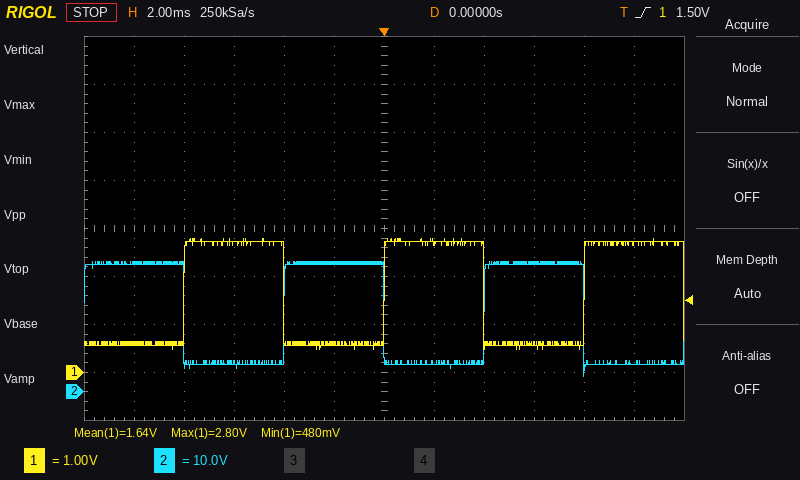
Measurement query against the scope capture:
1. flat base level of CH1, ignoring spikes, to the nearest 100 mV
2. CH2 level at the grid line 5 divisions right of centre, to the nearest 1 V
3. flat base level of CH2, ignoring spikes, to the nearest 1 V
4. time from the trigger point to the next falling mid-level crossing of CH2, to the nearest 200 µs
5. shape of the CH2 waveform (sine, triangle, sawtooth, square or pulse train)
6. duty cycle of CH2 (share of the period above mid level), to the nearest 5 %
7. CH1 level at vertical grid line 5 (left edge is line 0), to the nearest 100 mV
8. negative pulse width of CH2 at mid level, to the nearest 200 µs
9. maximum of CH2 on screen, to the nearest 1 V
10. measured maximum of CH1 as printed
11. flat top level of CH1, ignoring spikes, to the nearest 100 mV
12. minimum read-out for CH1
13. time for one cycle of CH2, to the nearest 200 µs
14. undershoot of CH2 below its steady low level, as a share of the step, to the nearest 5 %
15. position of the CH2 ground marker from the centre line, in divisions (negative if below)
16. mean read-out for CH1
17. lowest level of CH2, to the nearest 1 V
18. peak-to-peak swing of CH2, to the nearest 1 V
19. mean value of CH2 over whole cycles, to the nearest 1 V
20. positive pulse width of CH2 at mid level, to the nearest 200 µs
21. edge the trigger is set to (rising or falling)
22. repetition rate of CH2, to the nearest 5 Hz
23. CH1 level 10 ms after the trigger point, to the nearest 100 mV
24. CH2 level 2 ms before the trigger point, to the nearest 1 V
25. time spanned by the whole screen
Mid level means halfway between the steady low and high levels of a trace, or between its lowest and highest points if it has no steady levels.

600 mV
6 V
6 V
8.0 ms
square
50 %
600 mV
4.0 ms
27 V
2.80 V
2.7 V
480 mV
8.0 ms
10 %
-3.4 div
1.64 V
3 V
24 V
16 V
4.0 ms
rising
125 Hz
2.7 V
27 V
24 ms
